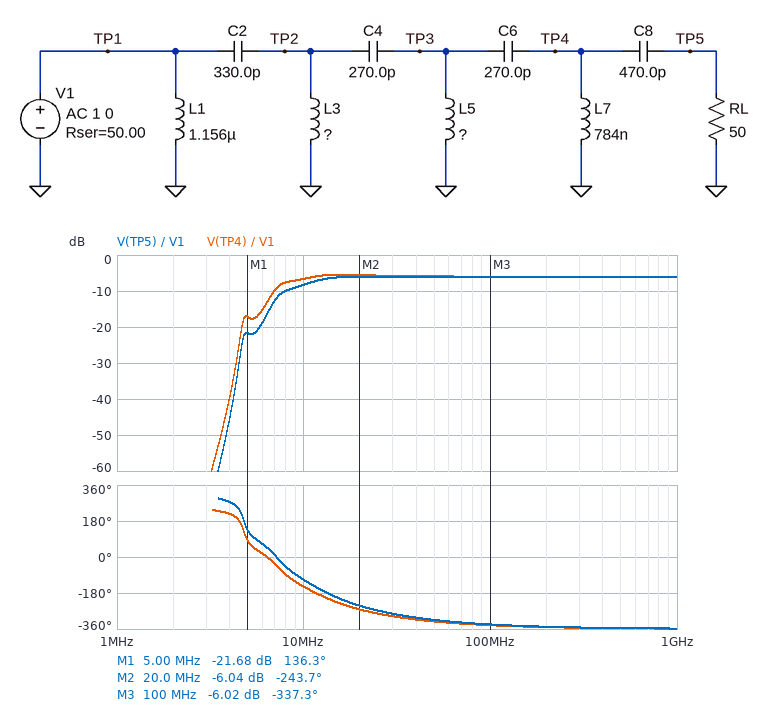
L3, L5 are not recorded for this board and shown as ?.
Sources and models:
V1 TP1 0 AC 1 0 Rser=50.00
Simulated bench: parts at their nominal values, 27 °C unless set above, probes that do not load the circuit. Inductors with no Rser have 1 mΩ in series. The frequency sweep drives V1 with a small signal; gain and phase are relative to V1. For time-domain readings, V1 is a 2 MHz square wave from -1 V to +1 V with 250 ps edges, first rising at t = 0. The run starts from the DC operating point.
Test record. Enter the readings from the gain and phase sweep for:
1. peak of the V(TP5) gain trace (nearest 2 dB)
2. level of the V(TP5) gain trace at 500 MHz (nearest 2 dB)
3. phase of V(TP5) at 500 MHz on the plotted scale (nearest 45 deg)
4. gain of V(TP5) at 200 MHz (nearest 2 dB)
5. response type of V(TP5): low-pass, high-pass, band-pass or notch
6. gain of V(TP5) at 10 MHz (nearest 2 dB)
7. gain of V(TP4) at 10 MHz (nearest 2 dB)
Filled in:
-6 dB
-6 dB
-360 deg
-6 dB
high-pass
-8 dB
-6 dB
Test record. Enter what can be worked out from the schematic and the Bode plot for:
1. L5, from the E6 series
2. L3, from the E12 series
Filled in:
470 nH
1.5 µH
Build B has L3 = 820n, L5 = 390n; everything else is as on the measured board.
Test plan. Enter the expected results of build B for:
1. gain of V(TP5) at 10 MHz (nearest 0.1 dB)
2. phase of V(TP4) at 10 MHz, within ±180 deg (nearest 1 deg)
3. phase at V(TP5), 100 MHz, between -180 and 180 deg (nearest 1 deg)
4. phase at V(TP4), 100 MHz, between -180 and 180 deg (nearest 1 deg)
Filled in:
-8.2 dB
-127 deg
25 deg
21 deg
